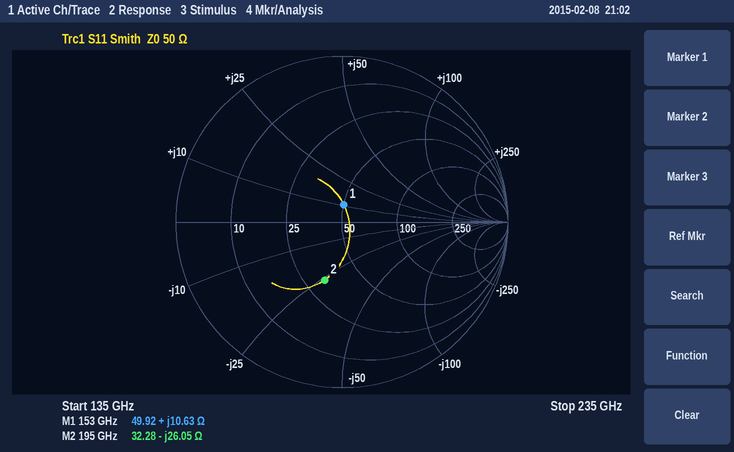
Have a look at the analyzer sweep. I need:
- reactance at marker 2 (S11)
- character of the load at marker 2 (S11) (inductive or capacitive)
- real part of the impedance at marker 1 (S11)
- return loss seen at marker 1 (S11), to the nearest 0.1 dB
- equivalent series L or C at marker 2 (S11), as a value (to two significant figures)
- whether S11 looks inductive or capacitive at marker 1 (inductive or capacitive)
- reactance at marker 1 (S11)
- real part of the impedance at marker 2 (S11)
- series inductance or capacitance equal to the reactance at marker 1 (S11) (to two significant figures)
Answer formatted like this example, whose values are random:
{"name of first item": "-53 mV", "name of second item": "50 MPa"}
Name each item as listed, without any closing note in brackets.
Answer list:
{"reactance at marker 2": "-26.05 Ω", "character of the load at marker 2 (S11)": "capacitive", "real part of the impedance at marker 1": "49.92 Ω", "return loss seen at marker 1 (S11), to the nearest 0.1 dB": "19.5 dB", "equivalent series L or C at marker 2 (S11), as a value": "31 fF", "whether S11 looks inductive or capacitive at marker 1": "inductive", "reactance at marker 1": "+10.63 Ω", "real part of the impedance at marker 2": "32.28 Ω", "series inductance or capacitance equal to the reactance at marker 1 (S11)": "11 pH"}
